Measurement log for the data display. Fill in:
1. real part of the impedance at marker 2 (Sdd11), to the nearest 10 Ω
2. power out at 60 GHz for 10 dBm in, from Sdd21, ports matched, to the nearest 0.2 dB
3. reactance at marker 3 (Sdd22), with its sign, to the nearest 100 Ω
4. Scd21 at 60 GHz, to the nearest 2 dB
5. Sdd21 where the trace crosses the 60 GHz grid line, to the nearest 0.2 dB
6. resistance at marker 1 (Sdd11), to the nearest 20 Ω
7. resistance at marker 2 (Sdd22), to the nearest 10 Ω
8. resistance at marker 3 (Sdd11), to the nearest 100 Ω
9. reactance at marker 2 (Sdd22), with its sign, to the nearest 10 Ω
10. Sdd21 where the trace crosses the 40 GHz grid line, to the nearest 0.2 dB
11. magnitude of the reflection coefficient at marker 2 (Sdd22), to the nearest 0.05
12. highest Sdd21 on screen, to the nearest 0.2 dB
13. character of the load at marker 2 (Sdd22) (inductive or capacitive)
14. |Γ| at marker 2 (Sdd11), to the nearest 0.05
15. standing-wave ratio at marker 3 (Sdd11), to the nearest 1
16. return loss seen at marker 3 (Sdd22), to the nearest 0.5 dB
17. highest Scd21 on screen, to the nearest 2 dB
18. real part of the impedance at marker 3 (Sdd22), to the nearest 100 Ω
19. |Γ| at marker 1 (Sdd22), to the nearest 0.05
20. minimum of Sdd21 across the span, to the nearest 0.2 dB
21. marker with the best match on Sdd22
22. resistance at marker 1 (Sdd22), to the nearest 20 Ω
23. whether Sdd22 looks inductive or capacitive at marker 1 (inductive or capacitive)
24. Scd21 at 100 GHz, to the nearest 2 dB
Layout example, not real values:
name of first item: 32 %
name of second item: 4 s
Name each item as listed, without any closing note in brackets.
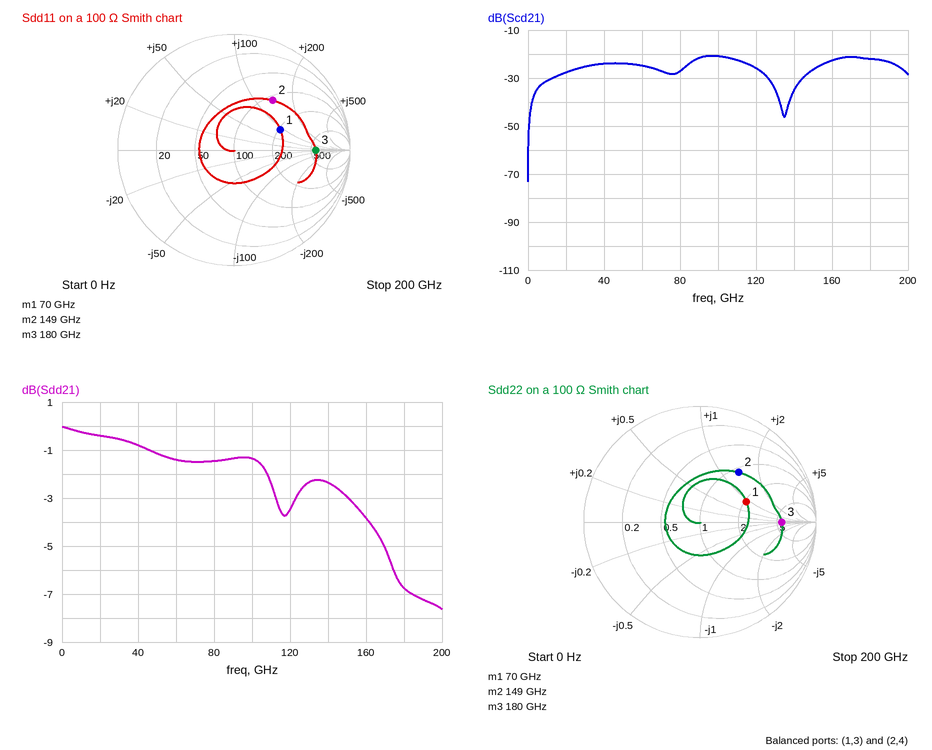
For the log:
real part of the impedance at marker 2 (Sdd11), to the nearest 10 Ω: 110 Ω
power out at 60 GHz for 10 dBm in, from Sdd21, ports matched, to the nearest 0.2 dB: 8.6 dBm
reactance at marker 3 (Sdd22), with its sign, to the nearest 100 Ω: 0 Ω
Scd21 at 60 GHz, to the nearest 2 dB: -24 dB
Sdd21 where the trace crosses the 60 GHz grid line, to the nearest 0.2 dB: -1.4 dB
resistance at marker 1 (Sdd11), to the nearest 20 Ω: 200 Ω
resistance at marker 2 (Sdd22), to the nearest 10 Ω: 110 Ω
resistance at marker 3 (Sdd11), to the nearest 100 Ω: 600 Ω
reactance at marker 2 (Sdd22), with its sign, to the nearest 10 Ω: +140 Ω
Sdd21 where the trace crosses the 40 GHz grid line, to the nearest 0.2 dB: -0.8 dB
magnitude of the reflection coefficient at marker 2 (Sdd22), to the nearest 0.05: 0.55
highest Sdd21 on screen, to the nearest 0.2 dB: 0.0 dB
character of the load at marker 2 (Sdd22): inductive
|Γ| at marker 2 (Sdd11), to the nearest 0.05: 0.55
standing-wave ratio at marker 3 (Sdd11), to the nearest 1: 6
return loss seen at marker 3 (Sdd22), to the nearest 0.5 dB: 3.0 dB
highest Scd21 on screen, to the nearest 2 dB: -20 dB
real part of the impedance at marker 3 (Sdd22), to the nearest 100 Ω: 600 Ω
|Γ| at marker 1 (Sdd22), to the nearest 0.05: 0.45
minimum of Sdd21 across the span, to the nearest 0.2 dB: -7.6 dB
marker with the best match on Sdd22: marker 1
resistance at marker 1 (Sdd22), to the nearest 20 Ω: 200 Ω
whether Sdd22 looks inductive or capacitive at marker 1: inductive
Scd21 at 100 GHz, to the nearest 2 dB: -20 dB
